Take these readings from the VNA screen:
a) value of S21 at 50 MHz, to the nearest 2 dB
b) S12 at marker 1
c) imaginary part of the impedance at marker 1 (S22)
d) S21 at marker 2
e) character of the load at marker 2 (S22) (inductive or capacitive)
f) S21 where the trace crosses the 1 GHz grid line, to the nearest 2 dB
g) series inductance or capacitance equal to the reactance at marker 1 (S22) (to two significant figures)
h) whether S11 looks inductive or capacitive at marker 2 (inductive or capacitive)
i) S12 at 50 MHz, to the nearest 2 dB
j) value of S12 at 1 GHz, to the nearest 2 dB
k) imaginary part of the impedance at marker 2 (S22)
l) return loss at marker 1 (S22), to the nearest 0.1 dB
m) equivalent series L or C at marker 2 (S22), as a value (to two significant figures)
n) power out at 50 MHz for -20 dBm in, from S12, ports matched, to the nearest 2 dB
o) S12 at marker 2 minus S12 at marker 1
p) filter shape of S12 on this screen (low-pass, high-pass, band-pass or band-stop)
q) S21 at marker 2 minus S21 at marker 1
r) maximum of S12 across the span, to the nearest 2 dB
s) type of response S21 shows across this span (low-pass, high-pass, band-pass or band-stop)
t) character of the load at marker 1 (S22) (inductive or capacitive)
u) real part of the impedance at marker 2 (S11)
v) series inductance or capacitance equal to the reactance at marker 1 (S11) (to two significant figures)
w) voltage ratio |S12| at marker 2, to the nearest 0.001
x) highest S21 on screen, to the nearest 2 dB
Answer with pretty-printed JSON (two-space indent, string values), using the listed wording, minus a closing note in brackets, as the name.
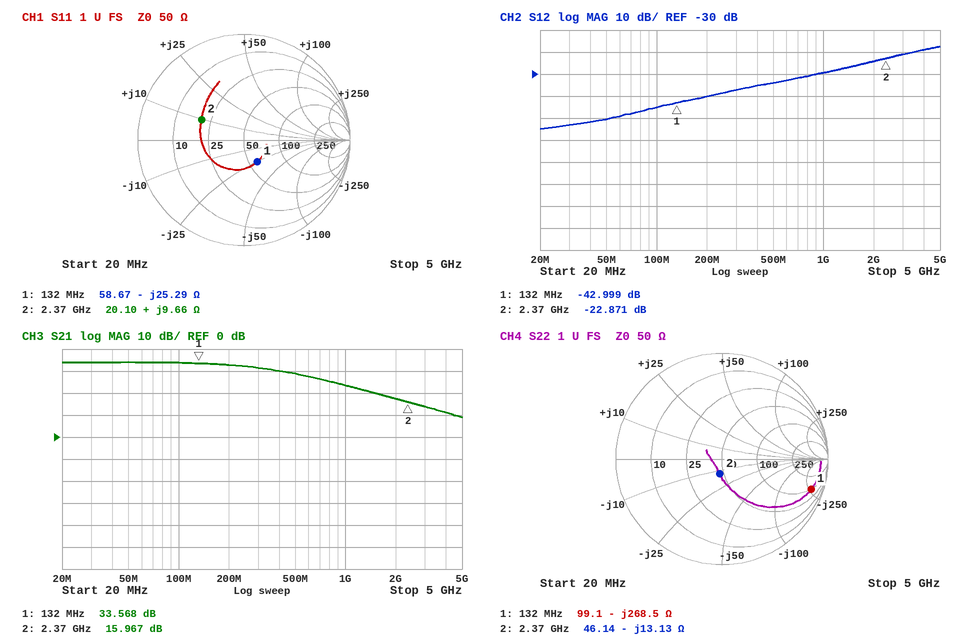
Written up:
{
  "value of S21 at 50 MHz, to the nearest 2 dB": "34 dB",
  "S12 at marker 1": "-42.999 dB",
  "imaginary part of the impedance at marker 1": "-268.5 Ω",
  "S21 at marker 2": "15.967 dB",
  "character of the load at marker 2 (S22)": "capacitive",
  "S21 where the trace crosses the 1 GHz grid line, to the nearest 2 dB": "24 dB",
  "series inductance or capacitance equal to the reactance at marker 1 (S22)": "4.5 pF",
  "whether S11 looks inductive or capacitive at marker 2": "inductive",
  "S12 at 50 MHz, to the nearest 2 dB": "-50 dB",
  "value of S12 at 1 GHz, to the nearest 2 dB": "-30 dB",
  "imaginary part of the impedance at marker 2": "-13.13 Ω",
  "return loss at marker 1 (S22), to the nearest 0.1 dB": "1.0 dB",
  "equivalent series L or C at marker 2 (S22), as a value": "5.1 pF",
  "power out at 50 MHz for -20 dBm in, from S12, ports matched, to the nearest 2 dB": "-70 dBm",
  "S12 at marker 2 minus S12 at marker 1": "20.128 dB",
  "filter shape of S12 on this screen": "high-pass",
  "S21 at marker 2 minus S21 at marker 1": "-17.601 dB",
  "maximum of S12 across the span, to the nearest 2 dB": "-18 dB",
  "type of response S21 shows across this span": "low-pass",
  "character of the load at marker 1 (S22)": "capacitive",
  "real part of the impedance at marker 2": "20.10 Ω",
  "series inductance or capacitance equal to the reactance at marker 1 (S11)": "48 pF",
  "voltage ratio |S12| at marker 2, to the nearest 0.001": "0.072",
  "highest S21 on screen, to the nearest 2 dB": "34 dB"
}
